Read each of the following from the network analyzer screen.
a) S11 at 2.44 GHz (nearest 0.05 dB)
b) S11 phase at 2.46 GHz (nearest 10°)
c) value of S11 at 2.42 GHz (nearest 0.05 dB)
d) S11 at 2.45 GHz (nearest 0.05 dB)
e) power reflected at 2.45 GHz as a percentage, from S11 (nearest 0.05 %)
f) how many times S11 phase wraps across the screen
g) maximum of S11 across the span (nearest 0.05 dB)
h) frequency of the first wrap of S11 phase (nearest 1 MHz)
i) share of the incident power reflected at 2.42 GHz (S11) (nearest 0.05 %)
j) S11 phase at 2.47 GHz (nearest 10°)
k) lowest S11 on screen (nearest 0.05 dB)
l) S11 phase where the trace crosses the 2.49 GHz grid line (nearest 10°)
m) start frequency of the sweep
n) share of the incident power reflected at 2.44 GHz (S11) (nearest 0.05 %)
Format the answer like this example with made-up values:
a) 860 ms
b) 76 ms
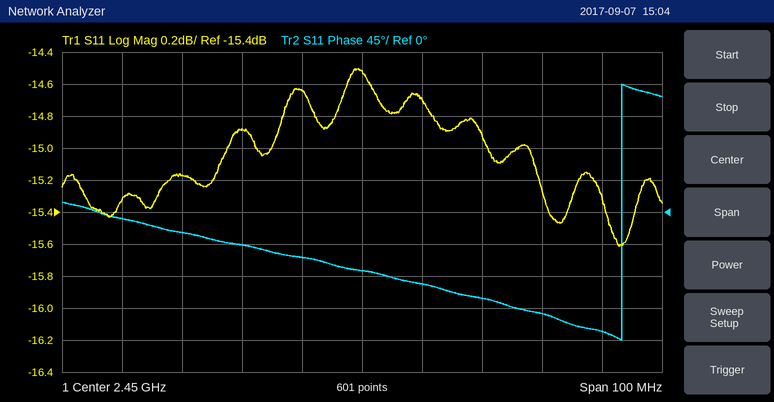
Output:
a) -14.65 dB
b) -100°
c) -15.15 dB
d) -14.50 dB
e) 3.55 %
f) 1
g) -14.50 dB
h) 2.493 GHz
i) 3.05 %
j) -120°
k) -15.60 dB
l) -170°
m) 2.4 GHz
n) 3.45 %
